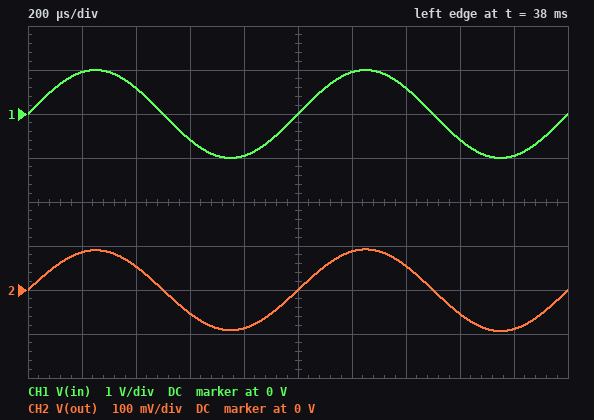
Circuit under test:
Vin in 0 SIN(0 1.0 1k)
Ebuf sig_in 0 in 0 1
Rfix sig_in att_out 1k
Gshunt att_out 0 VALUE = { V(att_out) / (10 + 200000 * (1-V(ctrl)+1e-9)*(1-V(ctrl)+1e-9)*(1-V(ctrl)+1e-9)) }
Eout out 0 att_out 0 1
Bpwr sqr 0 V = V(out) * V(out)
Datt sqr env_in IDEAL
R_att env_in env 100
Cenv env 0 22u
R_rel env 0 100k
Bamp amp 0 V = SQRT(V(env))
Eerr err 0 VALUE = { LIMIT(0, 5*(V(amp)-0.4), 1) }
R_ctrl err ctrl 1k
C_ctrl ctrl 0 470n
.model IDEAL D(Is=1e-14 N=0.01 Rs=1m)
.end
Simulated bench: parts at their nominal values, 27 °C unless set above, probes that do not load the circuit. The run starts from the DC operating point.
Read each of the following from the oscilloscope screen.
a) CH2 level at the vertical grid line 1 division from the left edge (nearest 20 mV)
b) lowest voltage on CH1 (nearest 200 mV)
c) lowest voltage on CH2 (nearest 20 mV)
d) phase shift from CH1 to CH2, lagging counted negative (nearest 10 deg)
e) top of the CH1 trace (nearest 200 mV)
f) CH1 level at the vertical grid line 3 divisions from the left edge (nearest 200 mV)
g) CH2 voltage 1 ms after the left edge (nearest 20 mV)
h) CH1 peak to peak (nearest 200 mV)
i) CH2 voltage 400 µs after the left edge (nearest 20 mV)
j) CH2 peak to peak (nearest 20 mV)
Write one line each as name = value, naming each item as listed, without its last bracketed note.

CH2 level at the vertical grid line 1 division from the left edge = 80 mV
lowest voltage on CH1 = -1.0 V
lowest voltage on CH2 = -100 mV
phase shift from CH1 to CH2, lagging counted negative = 0 deg
top of the CH1 trace = 1.0 V
CH1 level at the vertical grid line 3 divisions from the left edge = -600 mV
CH2 voltage 1 ms after the left edge = 0 V
CH1 peak to peak = 2.0 V
CH2 voltage 400 µs after the left edge = 60 mV
CH2 peak to peak = 180 mV
